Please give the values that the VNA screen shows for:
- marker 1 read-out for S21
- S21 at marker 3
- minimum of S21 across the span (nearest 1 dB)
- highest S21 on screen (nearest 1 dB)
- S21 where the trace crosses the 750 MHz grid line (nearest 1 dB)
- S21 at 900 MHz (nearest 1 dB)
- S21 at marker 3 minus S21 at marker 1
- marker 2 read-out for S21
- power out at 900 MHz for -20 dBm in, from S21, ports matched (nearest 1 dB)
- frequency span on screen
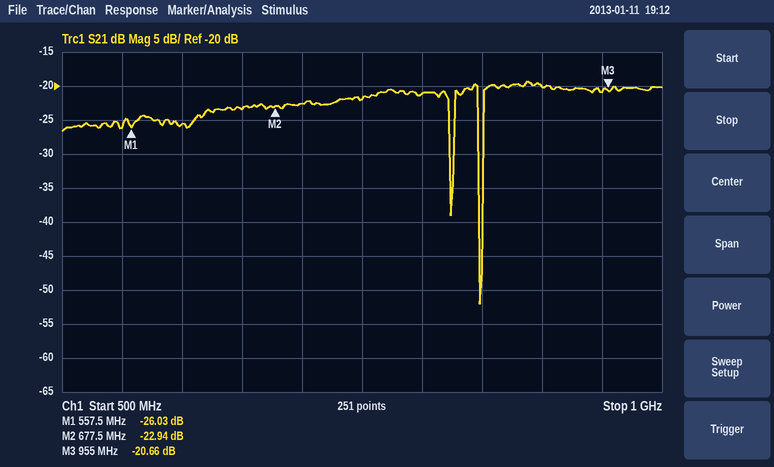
-26.03 dB
-20.66 dB
-52 dB
-19 dB
-22 dB
-20 dB
5.37 dB
-22.94 dB
-40 dBm
500 MHz
